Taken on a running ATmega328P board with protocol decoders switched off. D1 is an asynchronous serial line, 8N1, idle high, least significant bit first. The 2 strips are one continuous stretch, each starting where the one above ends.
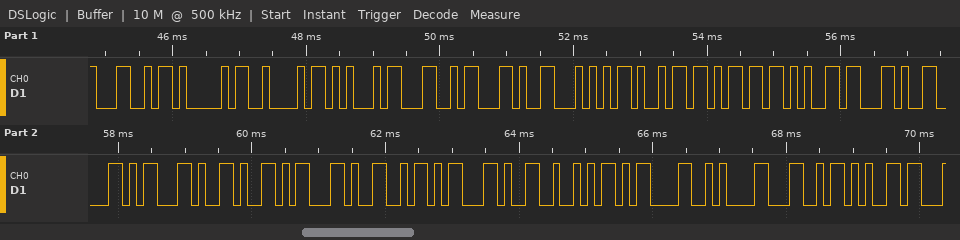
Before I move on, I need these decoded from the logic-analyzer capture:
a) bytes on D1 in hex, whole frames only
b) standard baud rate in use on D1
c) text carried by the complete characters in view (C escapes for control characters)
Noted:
4C 41 42 45 4C 2C 54 69 6D 65 2C 58 2C 59 2C 5A 2C 52 0D 0A 4C 65
9600 baud
"LABEL,Time,X,Y,Z,R\r\nLe"
